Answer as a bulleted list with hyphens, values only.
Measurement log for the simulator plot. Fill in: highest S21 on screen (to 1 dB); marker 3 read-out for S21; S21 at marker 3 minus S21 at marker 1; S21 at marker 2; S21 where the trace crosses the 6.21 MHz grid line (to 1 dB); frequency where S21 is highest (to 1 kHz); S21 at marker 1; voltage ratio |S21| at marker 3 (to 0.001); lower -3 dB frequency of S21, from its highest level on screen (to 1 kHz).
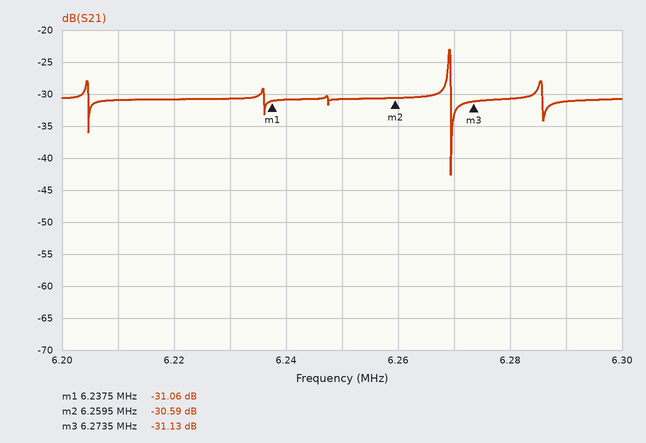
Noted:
- -23 dB
- -31.13 dB
- -0.07 dB
- -30.59 dB
- -31 dB
- 6.269 MHz
- -31.06 dB
- 0.028
- 6.269 MHz
